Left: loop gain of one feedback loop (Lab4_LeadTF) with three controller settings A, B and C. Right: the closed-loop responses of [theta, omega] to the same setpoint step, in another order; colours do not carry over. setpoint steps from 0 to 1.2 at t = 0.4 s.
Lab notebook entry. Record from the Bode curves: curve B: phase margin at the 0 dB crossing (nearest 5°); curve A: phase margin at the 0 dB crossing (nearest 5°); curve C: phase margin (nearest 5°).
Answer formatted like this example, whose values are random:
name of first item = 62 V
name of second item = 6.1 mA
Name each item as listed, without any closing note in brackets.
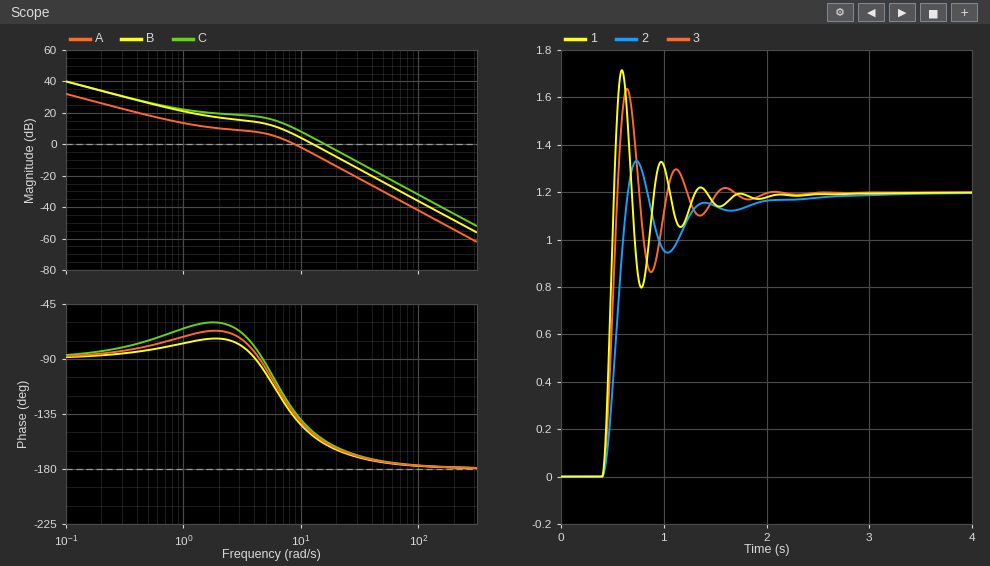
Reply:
curve B: phase margin at the 0 dB crossing = 25°
curve A: phase margin at the 0 dB crossing = 45°
curve C: phase margin = 25°
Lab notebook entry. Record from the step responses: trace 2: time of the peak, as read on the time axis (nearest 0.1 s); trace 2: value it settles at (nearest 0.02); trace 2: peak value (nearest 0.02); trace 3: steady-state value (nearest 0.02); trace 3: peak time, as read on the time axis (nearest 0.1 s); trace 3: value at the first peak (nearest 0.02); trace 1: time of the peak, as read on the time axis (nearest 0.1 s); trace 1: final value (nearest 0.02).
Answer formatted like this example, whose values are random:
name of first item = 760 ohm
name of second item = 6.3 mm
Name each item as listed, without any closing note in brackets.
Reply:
trace 2: time of the peak, as read on the time axis = 0.7 s
trace 2: value it settles at = 1.20
trace 2: peak value = 1.34
trace 3: steady-state value = 1.20
trace 3: peak time, as read on the time axis = 0.6 s
trace 3: value at the first peak = 1.64
trace 1: time of the peak, as read on the time axis = 0.6 s
trace 1: final value = 1.20
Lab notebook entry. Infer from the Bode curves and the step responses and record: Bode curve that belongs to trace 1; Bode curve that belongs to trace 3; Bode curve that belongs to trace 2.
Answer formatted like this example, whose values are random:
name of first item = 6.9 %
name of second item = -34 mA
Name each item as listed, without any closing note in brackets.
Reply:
Bode curve that belongs to trace 1 = C
Bode curve that belongs to trace 3 = B
Bode curve that belongs to trace 2 = A
